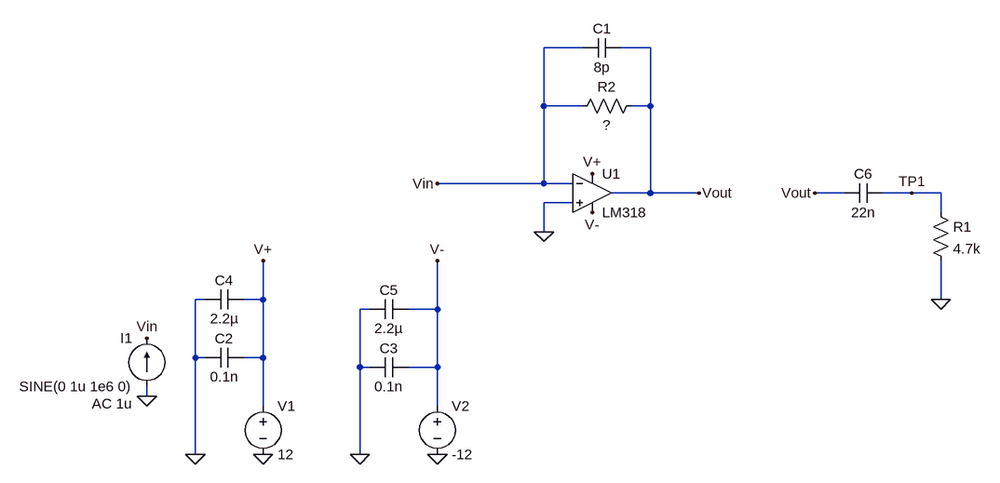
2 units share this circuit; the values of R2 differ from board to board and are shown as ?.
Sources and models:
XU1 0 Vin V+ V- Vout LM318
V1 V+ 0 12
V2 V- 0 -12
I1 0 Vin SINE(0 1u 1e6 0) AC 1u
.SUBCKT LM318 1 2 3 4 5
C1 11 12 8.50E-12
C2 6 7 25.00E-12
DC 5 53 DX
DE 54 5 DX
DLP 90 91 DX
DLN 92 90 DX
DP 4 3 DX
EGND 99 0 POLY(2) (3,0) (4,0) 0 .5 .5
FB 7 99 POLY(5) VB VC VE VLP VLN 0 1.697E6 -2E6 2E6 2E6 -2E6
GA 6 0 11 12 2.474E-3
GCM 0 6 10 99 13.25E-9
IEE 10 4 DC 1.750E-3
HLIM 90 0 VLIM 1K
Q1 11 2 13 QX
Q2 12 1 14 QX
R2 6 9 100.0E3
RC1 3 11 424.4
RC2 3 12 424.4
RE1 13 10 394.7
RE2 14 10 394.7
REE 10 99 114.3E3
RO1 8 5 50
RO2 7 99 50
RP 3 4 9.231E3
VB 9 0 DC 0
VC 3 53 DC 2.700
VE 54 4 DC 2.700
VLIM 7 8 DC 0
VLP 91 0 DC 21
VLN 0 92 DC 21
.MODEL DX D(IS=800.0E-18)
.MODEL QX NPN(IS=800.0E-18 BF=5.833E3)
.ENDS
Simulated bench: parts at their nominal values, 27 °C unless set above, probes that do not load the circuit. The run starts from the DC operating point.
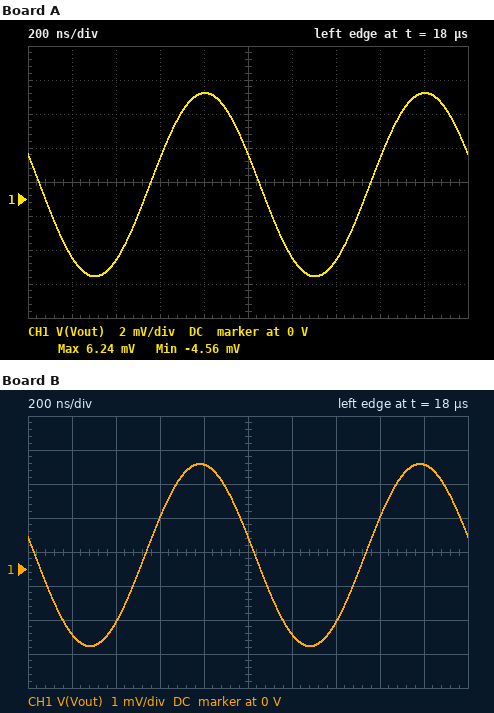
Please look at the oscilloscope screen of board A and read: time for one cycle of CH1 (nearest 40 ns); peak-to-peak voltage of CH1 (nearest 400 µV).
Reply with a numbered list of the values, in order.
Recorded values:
1. 1.00 µs
2. 10.8 mV
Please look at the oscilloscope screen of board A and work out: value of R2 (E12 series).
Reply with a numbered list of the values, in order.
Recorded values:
1. 5.6 kΩ
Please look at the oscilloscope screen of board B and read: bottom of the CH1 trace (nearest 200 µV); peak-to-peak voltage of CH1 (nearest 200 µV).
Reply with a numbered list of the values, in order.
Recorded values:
1. -2.2 mV
2. 5.4 mV
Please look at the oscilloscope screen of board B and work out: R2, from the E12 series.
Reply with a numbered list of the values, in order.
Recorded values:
1. 2.7 kΩ
